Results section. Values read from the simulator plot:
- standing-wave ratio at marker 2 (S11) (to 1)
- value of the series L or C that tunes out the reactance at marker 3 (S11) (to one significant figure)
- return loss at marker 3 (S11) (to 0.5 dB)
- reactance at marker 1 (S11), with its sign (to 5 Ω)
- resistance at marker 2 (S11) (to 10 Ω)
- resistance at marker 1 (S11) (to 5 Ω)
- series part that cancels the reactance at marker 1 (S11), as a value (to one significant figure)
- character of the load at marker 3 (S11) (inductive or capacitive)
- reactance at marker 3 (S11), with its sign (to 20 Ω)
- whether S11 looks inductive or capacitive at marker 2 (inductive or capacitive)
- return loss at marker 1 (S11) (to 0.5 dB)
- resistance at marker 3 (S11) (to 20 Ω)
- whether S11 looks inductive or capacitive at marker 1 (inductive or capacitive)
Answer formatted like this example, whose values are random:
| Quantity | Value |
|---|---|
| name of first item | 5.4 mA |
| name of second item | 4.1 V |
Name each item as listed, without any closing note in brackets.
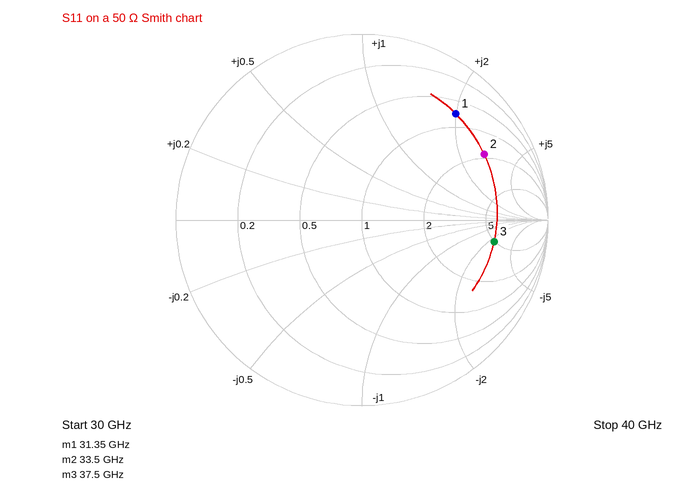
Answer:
| Quantity | Value |
|---|---|
| standing-wave ratio at marker 2 (S11) | 7 |
| value of the series L or C that tunes out the reactance at marker 3 (S11) | 500 pH |
| return loss at marker 3 (S11) | 3.0 dB |
| reactance at marker 1 (S11), with its sign | +100 Ω |
| resistance at marker 2 (S11) | 90 Ω |
| resistance at marker 1 (S11) | 35 Ω |
| series part that cancels the reactance at marker 1 (S11), as a value | 50 fF |
| character of the load at marker 3 (S11) | capacitive |
| reactance at marker 3 (S11), with its sign | -120 Ω |
| whether S11 looks inductive or capacitive at marker 2 | inductive |
| return loss at marker 1 (S11) | 2.5 dB |
| resistance at marker 3 (S11) | 240 Ω |
| whether S11 looks inductive or capacitive at marker 1 | inductive |
